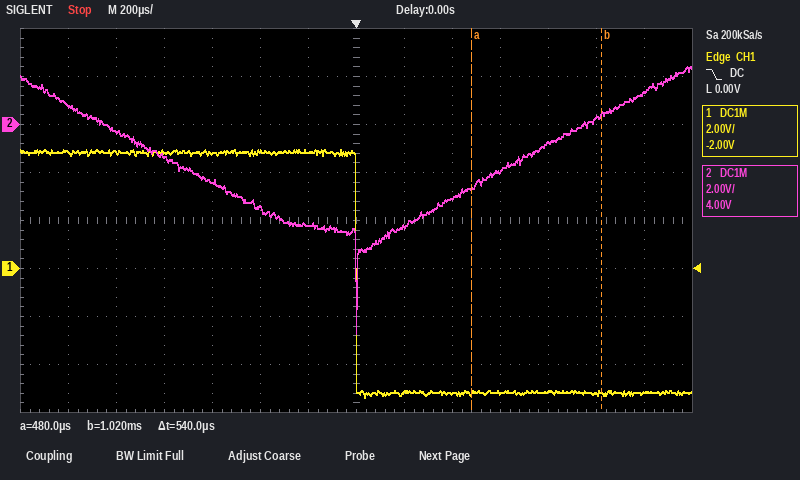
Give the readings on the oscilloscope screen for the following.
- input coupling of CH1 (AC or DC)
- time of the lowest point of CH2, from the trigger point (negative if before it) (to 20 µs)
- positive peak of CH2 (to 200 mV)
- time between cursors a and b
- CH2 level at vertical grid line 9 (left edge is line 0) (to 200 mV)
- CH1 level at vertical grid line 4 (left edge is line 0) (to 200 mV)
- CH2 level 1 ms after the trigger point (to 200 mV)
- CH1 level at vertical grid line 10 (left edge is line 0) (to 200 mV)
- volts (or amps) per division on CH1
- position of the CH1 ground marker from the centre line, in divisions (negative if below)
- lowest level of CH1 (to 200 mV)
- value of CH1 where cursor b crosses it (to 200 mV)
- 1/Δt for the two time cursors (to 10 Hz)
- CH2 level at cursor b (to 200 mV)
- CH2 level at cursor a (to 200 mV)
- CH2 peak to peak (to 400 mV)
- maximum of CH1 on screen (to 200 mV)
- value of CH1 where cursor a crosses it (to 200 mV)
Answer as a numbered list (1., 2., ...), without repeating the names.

1. DC
2. 0 µs
3. 2.4 V
4. 540 µs
5. -3.0 V
6. 4.8 V
7. 200 mV
8. -5.2 V
9. 2 V
10. -1.0 div
11. -5.4 V
12. -5.2 V
13. 1.85 kHz
14. 400 mV
15. -2.6 V
16. 11.2 V
17. 5.0 V
18. -5.2 V
